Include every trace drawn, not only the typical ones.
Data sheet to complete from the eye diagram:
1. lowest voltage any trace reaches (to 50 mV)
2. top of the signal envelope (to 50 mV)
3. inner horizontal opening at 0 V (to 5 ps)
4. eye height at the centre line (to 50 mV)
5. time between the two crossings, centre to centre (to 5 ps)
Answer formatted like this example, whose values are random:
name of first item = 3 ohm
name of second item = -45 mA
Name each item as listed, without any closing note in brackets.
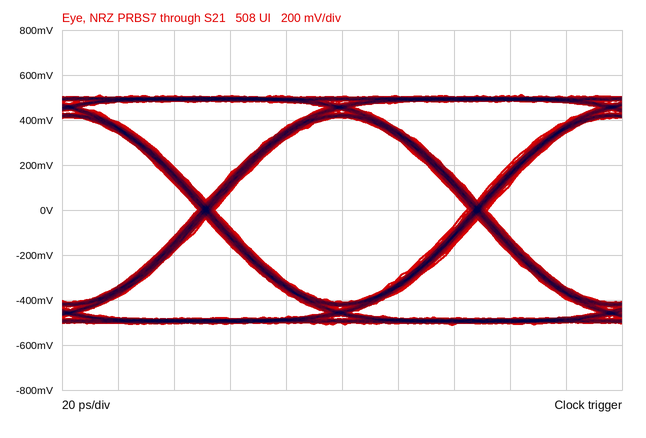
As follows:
lowest voltage any trace reaches = -500 mV
top of the signal envelope = 500 mV
inner horizontal opening at 0 V = 90 ps
eye height at the centre line = 800 mV
time between the two crossings, centre to centre = 95 ps
